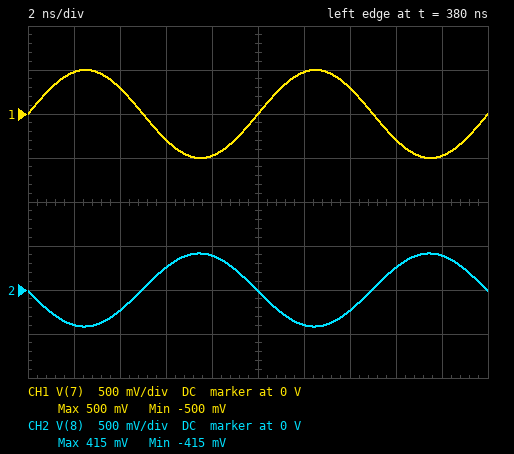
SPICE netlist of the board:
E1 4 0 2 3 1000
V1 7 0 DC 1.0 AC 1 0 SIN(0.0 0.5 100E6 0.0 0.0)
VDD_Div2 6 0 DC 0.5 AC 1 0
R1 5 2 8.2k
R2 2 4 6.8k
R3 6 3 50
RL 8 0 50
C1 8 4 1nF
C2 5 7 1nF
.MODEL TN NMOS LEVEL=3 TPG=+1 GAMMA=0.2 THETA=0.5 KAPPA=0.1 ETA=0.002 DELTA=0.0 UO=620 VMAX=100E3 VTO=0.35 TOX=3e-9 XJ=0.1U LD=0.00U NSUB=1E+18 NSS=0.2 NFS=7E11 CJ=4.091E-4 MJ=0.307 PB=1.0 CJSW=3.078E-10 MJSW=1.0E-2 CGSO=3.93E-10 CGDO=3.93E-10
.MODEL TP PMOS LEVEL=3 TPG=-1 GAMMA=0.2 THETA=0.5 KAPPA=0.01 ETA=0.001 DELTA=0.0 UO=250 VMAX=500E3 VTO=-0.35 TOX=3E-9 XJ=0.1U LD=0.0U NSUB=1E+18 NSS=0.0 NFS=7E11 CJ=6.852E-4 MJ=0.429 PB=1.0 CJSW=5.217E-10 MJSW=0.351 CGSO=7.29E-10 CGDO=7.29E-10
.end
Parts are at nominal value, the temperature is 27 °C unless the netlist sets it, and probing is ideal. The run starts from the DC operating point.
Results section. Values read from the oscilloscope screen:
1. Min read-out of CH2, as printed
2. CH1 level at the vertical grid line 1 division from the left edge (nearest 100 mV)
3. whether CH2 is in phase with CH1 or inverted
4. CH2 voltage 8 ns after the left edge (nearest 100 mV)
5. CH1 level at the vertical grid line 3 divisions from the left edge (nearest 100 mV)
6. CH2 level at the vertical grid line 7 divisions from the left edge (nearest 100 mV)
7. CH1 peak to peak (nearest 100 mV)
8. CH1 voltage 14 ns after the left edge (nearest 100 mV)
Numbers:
-415 mV
500 mV
inverted
400 mV
-300 mV
-200 mV
1.0 V
300 mV
